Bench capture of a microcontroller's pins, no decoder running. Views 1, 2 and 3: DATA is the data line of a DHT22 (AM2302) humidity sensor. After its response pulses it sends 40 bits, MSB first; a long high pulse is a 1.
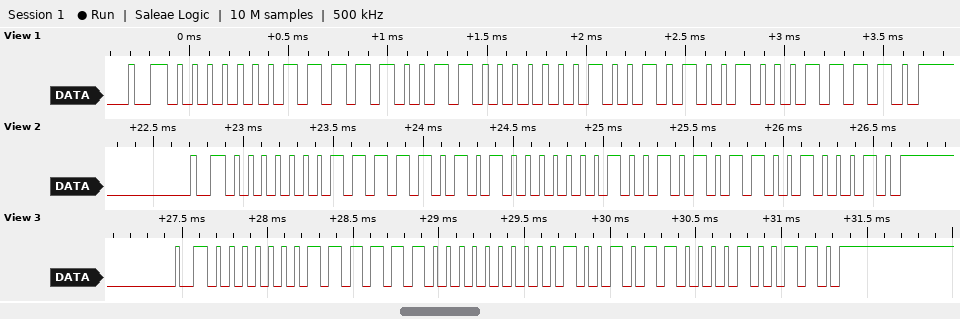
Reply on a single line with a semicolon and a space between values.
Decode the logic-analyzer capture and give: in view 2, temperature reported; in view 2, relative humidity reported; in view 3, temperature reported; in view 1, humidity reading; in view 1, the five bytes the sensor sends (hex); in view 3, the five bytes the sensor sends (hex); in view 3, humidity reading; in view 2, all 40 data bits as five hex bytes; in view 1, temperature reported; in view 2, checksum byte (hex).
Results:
29.9 °C; 50.1 %; 30.0 °C; 49.9 %; 01 F3 01 29 1E; 01 F8 01 2C 26; 50.4 %; 01 F5 01 2B 22; 29.7 °C; 0x22
